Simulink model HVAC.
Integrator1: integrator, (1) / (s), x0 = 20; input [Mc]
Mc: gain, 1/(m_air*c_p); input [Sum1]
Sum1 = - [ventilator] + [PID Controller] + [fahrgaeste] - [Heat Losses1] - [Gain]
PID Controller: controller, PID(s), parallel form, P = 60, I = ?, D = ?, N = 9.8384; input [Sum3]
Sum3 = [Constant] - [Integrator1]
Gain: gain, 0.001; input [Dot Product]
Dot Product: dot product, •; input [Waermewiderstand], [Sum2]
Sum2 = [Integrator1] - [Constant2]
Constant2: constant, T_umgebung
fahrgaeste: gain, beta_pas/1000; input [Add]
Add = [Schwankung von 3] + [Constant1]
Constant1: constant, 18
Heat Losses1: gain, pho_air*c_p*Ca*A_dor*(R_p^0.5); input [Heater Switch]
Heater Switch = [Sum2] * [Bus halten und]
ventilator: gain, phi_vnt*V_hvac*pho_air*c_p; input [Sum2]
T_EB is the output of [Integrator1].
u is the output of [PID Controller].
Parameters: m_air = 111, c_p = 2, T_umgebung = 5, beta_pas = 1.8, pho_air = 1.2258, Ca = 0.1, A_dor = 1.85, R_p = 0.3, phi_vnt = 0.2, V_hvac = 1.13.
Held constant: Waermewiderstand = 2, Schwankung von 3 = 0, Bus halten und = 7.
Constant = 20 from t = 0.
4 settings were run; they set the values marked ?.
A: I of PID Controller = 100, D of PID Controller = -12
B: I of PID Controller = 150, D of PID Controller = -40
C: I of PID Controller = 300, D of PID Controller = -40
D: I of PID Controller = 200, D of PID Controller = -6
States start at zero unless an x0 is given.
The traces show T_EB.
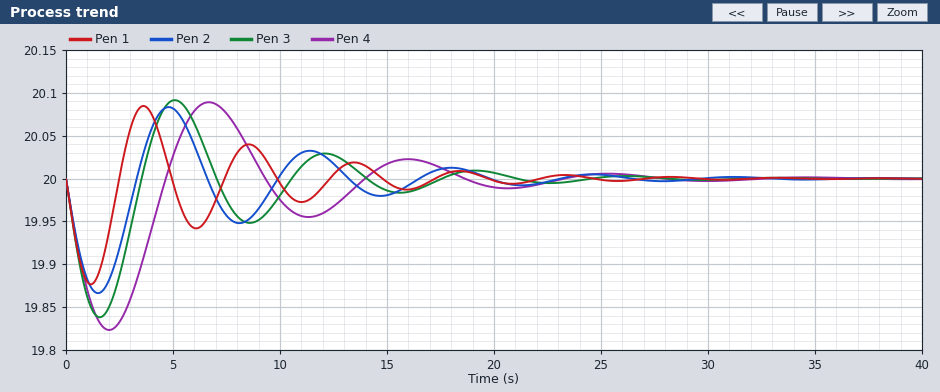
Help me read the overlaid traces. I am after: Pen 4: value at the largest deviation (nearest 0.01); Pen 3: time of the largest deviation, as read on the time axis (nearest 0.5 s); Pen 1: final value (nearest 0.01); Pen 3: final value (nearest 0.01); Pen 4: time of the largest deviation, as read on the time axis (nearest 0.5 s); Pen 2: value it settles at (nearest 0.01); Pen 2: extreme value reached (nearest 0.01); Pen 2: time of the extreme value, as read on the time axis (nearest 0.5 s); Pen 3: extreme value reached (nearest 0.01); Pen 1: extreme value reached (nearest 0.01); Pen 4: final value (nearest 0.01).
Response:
19.82
1.5 s
20.00
20.00
2.0 s
20.00
19.87
1.5 s
19.84
19.88
20.00
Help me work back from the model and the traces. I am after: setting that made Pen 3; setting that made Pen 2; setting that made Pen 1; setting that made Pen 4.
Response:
B
D
C
A
